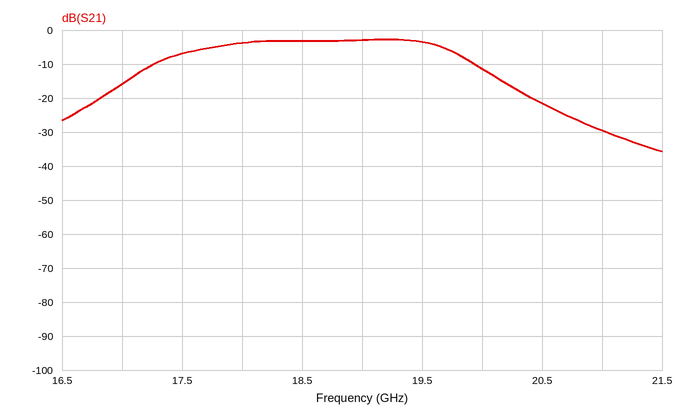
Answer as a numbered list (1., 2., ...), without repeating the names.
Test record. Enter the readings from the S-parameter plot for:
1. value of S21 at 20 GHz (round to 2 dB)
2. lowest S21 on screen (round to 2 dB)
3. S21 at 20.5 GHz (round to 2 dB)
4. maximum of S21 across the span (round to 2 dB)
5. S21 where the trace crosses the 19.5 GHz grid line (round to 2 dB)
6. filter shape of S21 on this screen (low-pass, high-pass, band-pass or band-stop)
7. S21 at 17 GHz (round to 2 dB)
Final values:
1. -12 dB
2. -36 dB
3. -22 dB
4. -2 dB
5. -4 dB
6. band-pass
7. -16 dB
